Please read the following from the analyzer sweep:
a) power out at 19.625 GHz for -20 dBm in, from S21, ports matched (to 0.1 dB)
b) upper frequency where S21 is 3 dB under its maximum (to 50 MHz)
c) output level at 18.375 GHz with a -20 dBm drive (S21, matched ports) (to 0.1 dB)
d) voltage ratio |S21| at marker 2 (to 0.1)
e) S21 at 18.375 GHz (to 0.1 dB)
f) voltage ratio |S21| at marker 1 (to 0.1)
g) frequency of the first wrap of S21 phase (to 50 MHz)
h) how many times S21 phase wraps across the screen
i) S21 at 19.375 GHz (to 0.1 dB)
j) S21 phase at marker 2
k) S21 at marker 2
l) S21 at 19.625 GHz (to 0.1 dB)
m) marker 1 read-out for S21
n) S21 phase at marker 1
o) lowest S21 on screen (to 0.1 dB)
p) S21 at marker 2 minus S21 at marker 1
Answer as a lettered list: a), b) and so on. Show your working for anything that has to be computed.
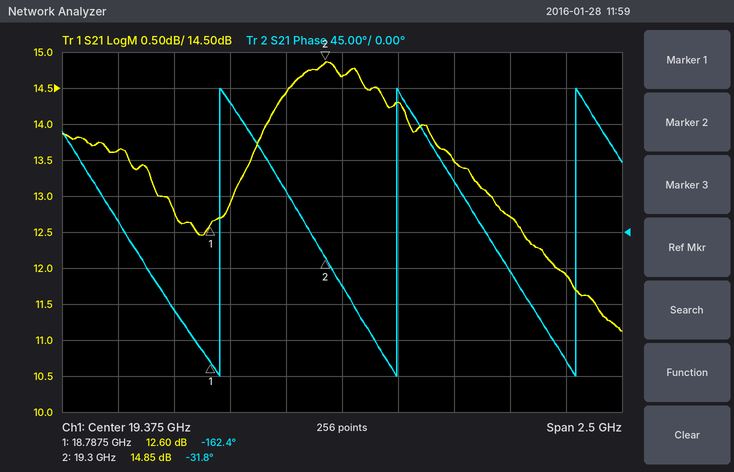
a) -20 dBm + (14.3 dB) = -5.7 dBm
b) 20.40 GHz
c) -20 dBm + (13.6 dB) = -6.4 dBm
d) 10^(14.85/20) ≈ 5.5
e) 13.6 dB
f) 10^(12.6/20) ≈ 4.3
g) 18.85 GHz
h) 3
i) 14.7 dB
j) -31.8°
k) 14.85 dB
l) 14.3 dB
m) 12.60 dB
n) -162.4°
o) 11.1 dB
p) 14.85 − (12.6) = 2.25 dB
